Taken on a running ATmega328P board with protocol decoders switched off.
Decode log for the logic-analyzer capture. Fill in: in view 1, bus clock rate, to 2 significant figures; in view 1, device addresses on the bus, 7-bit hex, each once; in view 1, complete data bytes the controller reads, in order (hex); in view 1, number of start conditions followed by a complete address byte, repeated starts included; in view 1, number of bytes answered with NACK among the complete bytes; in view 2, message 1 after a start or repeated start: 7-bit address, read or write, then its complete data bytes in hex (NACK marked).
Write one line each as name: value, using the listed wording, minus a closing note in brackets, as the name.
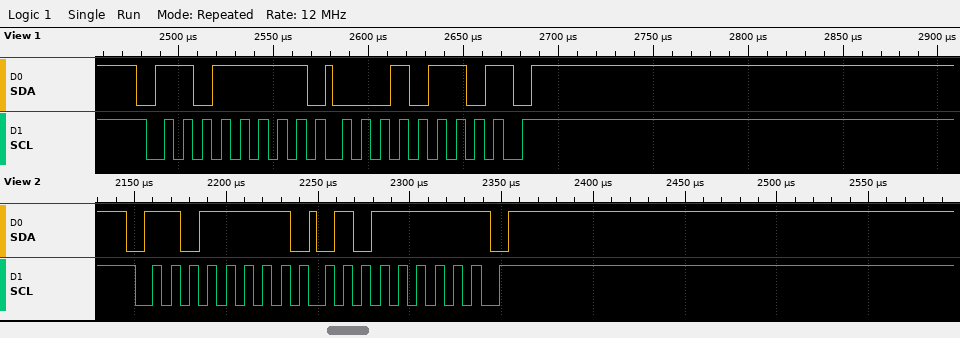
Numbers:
in view 1, bus clock rate, to 2 significant figures: 100 kHz
in view 1, device addresses on the bus, 7-bit hex, each once: 0x6F
in view 1, complete data bytes the controller reads, in order: 16
in view 1, number of start conditions followed by a complete address byte, repeated starts included: 1
in view 1, number of bytes answered with NACK among the complete bytes: 1
in view 2, message 1 after a start or repeated start: 7-bit address, read or write, then its complete data bytes in hex: 0x6F read: 5F NACK
